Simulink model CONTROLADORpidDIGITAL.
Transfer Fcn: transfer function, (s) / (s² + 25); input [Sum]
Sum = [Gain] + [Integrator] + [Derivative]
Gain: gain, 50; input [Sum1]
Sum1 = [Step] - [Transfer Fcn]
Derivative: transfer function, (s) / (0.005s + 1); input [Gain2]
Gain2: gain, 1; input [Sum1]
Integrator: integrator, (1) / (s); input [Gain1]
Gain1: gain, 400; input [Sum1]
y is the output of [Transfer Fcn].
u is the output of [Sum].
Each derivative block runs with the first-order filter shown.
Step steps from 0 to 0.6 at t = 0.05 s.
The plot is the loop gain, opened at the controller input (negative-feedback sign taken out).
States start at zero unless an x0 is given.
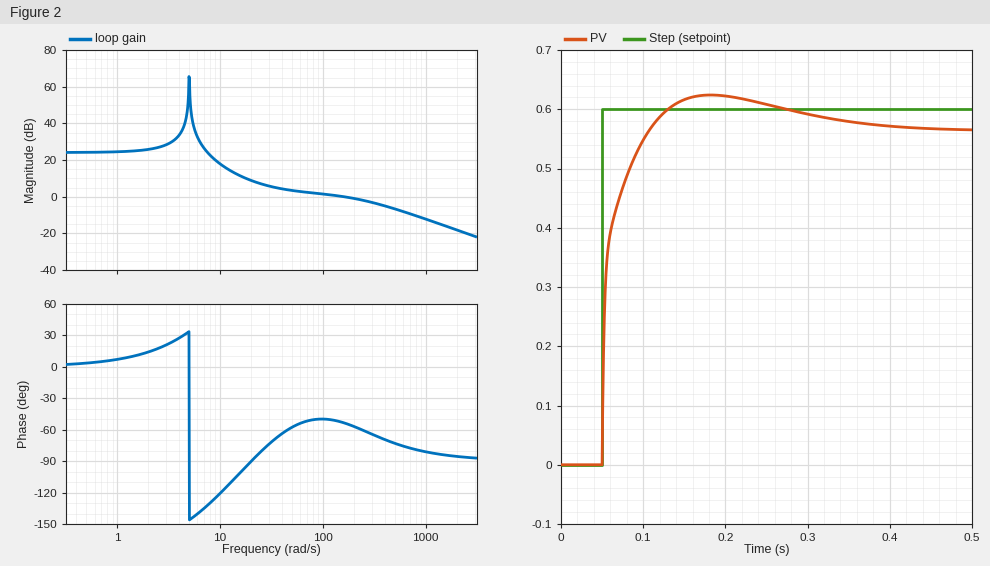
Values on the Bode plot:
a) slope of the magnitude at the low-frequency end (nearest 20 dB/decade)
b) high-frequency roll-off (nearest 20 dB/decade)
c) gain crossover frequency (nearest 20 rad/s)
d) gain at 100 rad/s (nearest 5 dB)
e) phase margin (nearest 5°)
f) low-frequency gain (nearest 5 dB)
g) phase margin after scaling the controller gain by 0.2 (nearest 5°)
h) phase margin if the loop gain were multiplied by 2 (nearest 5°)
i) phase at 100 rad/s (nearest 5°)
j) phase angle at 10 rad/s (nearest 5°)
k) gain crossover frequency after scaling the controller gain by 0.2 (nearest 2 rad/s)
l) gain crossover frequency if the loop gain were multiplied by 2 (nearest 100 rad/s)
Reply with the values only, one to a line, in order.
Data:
0 dB/decade
-20 dB/decade
160 rad/s
0 dB
125°
25 dB
70°
110°
-50°
-120°
12 rad/s
500 rad/s
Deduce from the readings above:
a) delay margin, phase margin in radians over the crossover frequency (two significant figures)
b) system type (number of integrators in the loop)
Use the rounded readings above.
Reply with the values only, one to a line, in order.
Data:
0.014 s
0
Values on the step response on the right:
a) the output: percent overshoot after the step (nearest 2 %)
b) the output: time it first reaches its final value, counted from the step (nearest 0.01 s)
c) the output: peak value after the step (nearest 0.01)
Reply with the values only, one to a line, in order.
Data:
10 %
0.06 s
0.62
